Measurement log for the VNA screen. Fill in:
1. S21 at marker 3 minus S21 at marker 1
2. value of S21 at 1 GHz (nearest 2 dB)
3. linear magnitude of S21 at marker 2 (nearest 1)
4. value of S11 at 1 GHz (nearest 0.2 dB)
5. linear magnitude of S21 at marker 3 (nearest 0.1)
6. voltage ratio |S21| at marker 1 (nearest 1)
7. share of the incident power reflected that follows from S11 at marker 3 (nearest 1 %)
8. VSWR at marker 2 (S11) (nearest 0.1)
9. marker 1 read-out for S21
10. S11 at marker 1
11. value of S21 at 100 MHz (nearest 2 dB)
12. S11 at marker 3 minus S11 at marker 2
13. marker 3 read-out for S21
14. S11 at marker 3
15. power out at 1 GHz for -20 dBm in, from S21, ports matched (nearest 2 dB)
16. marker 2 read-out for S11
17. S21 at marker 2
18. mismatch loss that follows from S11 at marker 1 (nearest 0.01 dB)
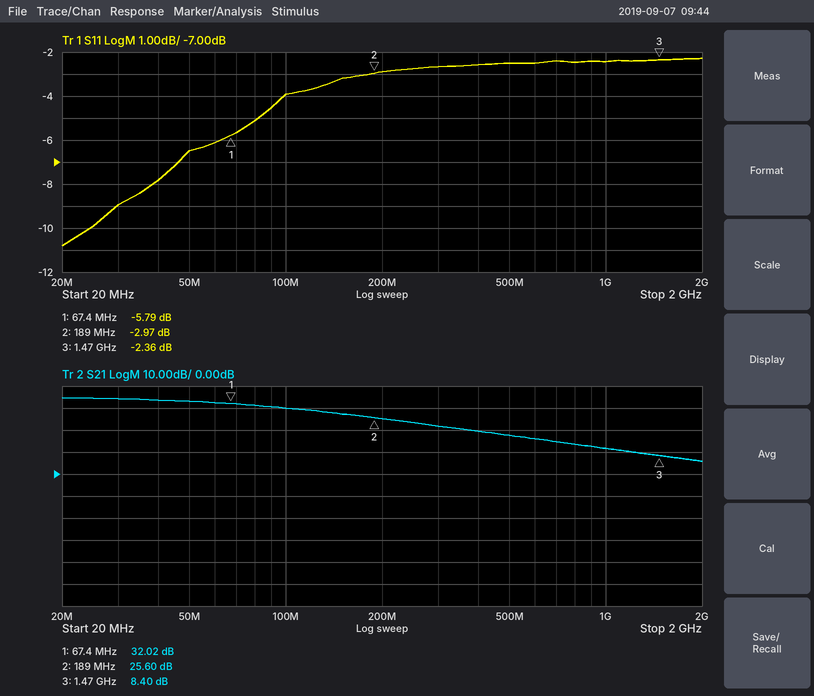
-23.62 dB
12 dB
19
-2.4 dB
2.6
40
58 %
5.9
32.02 dB
-5.79 dB
30 dB
0.61 dB
8.40 dB
-2.36 dB
-8 dBm
-2.97 dB
25.60 dB
1.33 dB
